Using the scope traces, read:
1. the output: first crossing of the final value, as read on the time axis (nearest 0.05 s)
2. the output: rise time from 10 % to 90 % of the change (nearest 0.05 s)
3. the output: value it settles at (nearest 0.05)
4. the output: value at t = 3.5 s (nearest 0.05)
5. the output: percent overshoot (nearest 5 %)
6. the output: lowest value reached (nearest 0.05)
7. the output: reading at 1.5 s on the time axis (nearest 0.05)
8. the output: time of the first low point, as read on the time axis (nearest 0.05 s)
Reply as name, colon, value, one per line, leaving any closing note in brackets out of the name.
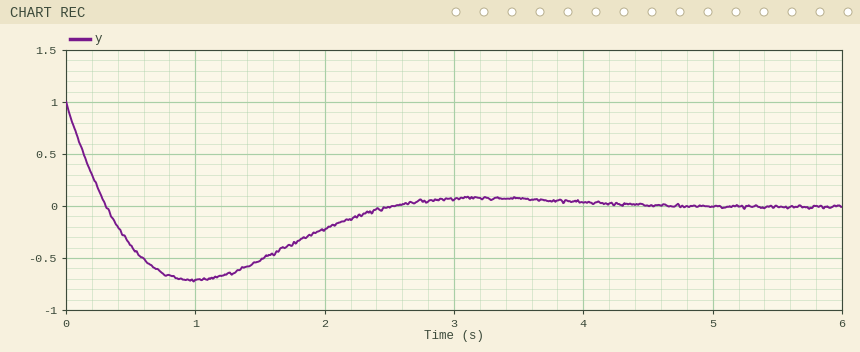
the output: first crossing of the final value, as read on the time axis: 0.30 s
the output: rise time from 10 % to 90 % of the change: 0.25 s
the output: value it settles at: 0.00
the output: value at t = 3.5 s: 0.05
the output: percent overshoot: 70 %
the output: lowest value reached: -0.70
the output: reading at 1.5 s on the time axis: -0.50
the output: time of the first low point, as read on the time axis: 1.00 s
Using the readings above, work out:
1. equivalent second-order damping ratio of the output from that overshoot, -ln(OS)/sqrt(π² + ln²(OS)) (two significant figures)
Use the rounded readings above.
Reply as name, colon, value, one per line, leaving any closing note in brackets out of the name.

equivalent second-order damping ratio of the output from that overshoot, -ln(OS)/sqrt(π² + ln²(OS)): 0.11
